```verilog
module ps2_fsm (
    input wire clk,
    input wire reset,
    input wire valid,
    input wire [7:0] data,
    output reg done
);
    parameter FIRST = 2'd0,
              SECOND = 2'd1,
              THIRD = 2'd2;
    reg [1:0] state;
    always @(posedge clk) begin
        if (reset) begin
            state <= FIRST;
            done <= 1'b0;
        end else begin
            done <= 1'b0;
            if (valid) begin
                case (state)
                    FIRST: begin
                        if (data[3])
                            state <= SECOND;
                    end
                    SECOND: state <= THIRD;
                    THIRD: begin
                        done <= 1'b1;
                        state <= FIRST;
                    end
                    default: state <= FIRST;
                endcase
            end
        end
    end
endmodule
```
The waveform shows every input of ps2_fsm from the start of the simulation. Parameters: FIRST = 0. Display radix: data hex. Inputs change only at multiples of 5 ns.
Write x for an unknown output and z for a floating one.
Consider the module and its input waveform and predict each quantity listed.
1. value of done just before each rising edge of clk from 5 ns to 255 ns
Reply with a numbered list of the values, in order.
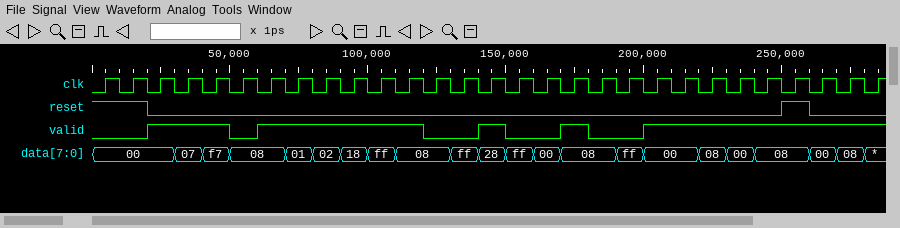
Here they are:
1. x 0 0 0 0 0 0 0 0 1 0 0 1 0 0 0 0 0 0 0 0 1 0 0 0 1
